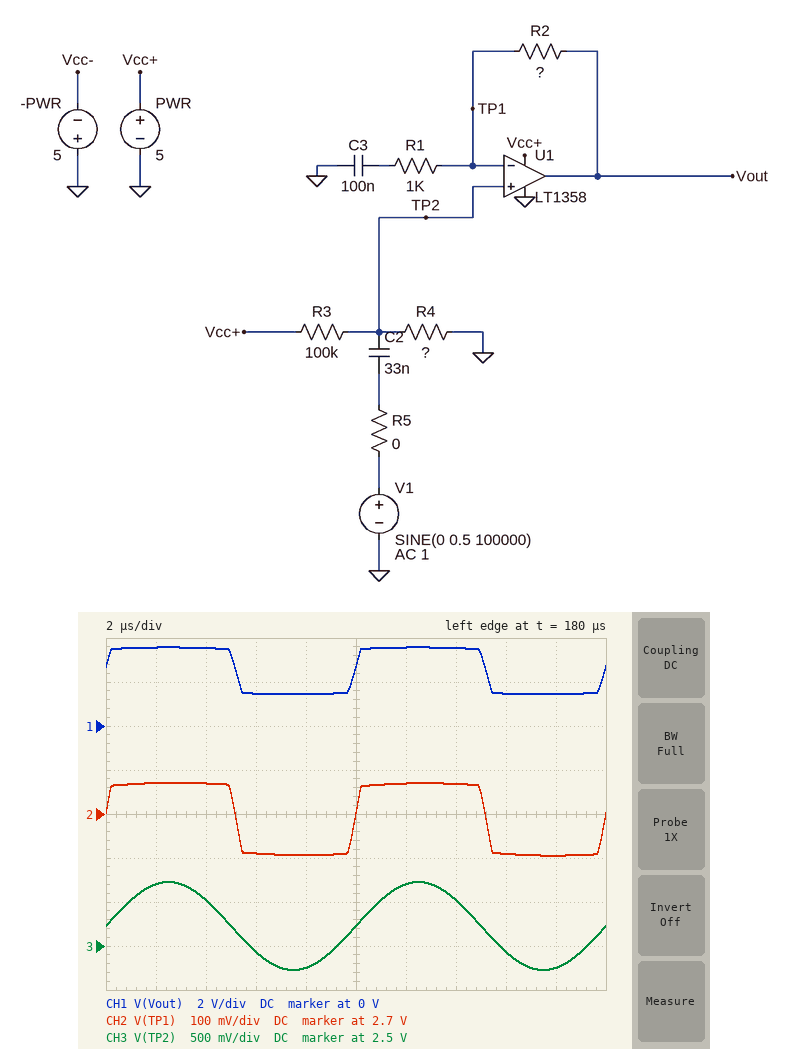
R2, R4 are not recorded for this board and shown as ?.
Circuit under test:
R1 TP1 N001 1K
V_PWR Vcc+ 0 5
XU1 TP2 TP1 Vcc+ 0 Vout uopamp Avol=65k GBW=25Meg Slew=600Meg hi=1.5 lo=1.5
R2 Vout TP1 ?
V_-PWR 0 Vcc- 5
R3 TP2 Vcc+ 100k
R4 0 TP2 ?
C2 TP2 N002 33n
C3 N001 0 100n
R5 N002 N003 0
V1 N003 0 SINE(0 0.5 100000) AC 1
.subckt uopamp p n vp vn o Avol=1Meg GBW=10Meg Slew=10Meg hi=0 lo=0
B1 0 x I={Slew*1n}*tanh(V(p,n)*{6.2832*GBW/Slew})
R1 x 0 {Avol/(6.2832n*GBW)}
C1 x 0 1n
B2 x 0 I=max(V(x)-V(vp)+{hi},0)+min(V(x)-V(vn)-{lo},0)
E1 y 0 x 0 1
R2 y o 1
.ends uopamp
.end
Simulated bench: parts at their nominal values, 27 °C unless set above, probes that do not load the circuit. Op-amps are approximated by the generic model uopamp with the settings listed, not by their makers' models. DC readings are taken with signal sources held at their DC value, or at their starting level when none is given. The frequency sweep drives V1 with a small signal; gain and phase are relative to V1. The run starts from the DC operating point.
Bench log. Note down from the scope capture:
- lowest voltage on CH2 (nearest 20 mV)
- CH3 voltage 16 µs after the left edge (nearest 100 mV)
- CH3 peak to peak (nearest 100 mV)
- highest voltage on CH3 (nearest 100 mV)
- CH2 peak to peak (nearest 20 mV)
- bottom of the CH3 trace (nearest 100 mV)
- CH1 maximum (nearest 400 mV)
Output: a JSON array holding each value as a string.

["2.60 V", "2.4 V", "1.0 V", "3.2 V", "160 mV", "2.2 V", "3.6 V"]
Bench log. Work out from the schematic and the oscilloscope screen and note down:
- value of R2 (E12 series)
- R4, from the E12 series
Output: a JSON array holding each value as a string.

["12 kΩ", "120 kΩ"]
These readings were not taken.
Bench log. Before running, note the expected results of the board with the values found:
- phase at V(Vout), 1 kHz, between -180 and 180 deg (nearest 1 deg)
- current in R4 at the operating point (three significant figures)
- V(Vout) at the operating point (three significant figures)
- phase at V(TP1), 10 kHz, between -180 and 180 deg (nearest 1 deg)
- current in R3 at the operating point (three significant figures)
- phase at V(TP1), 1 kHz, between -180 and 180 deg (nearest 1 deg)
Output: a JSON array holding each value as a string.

["56 deg", "22.7 µA", "2.73 V", "0 deg", "22.7 µA", "5 deg"]
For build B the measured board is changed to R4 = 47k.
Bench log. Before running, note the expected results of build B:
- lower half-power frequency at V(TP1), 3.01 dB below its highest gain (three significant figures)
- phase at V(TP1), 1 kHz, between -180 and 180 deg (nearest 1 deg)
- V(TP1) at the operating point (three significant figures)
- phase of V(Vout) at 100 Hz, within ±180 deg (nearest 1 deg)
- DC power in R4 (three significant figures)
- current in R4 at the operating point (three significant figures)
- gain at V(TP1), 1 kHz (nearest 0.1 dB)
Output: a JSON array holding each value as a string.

["151 Hz", "9 deg", "1.60 V", "92 deg", "54.4 µW", "34.0 µA", "-0.1 dB"]
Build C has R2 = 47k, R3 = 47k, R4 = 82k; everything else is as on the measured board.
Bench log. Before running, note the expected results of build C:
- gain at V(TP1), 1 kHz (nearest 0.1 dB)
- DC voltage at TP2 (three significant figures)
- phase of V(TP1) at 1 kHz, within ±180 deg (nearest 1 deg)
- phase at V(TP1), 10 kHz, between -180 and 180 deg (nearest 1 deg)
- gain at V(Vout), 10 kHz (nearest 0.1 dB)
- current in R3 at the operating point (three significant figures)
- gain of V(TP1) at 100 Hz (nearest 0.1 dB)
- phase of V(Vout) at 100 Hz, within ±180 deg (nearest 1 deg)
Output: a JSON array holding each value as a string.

["-0.1 dB", "3.18 V", "9 deg", "0 deg", "33.5 dB", "38.8 µA", "-5.6 dB", "126 deg"]
